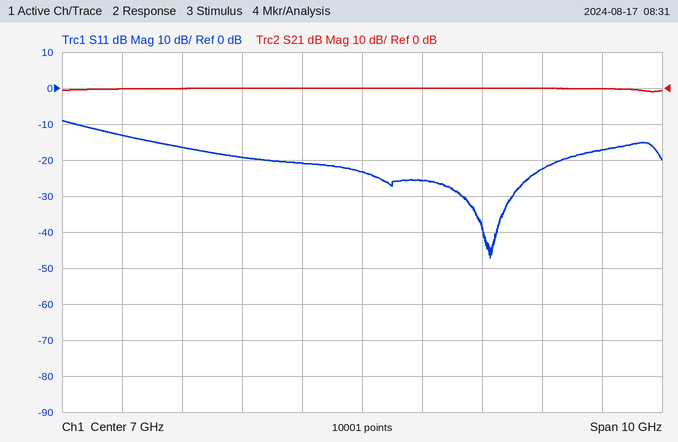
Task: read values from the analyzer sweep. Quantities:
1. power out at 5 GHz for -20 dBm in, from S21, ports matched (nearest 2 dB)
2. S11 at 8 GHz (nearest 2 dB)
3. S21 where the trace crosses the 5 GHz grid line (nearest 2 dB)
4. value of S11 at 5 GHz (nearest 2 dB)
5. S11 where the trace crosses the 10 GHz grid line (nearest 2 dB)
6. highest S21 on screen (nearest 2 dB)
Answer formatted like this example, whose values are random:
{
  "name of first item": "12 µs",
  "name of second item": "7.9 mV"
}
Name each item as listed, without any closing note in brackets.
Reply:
{
  "power out at 5 GHz for -20 dBm in, from S21, ports matched": "-20 dBm",
  "S11 at 8 GHz": "-26 dB",
  "S21 where the trace crosses the 5 GHz grid line": "0 dB",
  "value of S11 at 5 GHz": "-20 dB",
  "S11 where the trace crosses the 10 GHz grid line": "-22 dB",
  "highest S21 on screen": "0 dB"
}
